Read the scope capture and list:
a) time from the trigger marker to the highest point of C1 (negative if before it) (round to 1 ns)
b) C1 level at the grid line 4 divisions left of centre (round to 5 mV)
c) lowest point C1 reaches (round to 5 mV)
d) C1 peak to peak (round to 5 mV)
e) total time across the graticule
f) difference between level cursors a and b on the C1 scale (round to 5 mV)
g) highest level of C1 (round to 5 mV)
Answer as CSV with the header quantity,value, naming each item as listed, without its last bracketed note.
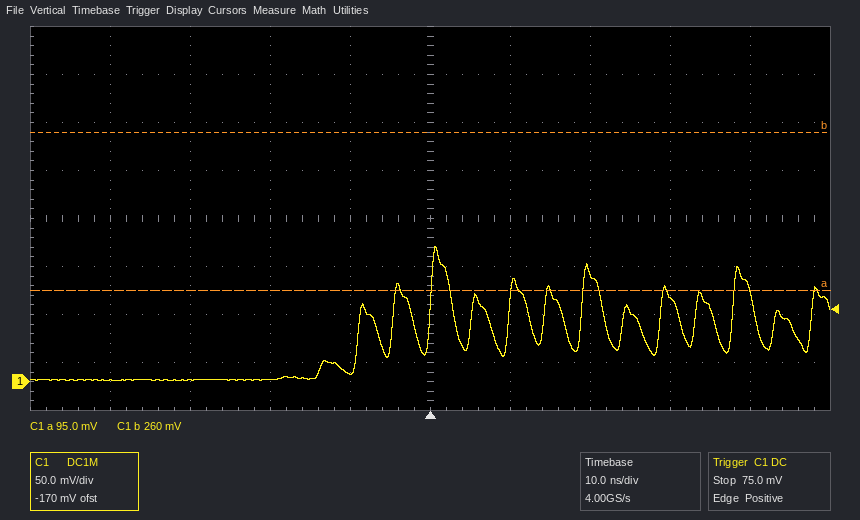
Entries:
quantity,value
time from the trigger marker to the highest point of C1 (negative if before it),+1 ns
C1 level at the grid line 4 divisions left of centre,0 mV
lowest point C1 reaches,0 mV
C1 peak to peak,140 mV
total time across the graticule,100 ns
difference between level cursors a and b on the C1 scale,165 mV
highest level of C1,140 mV
